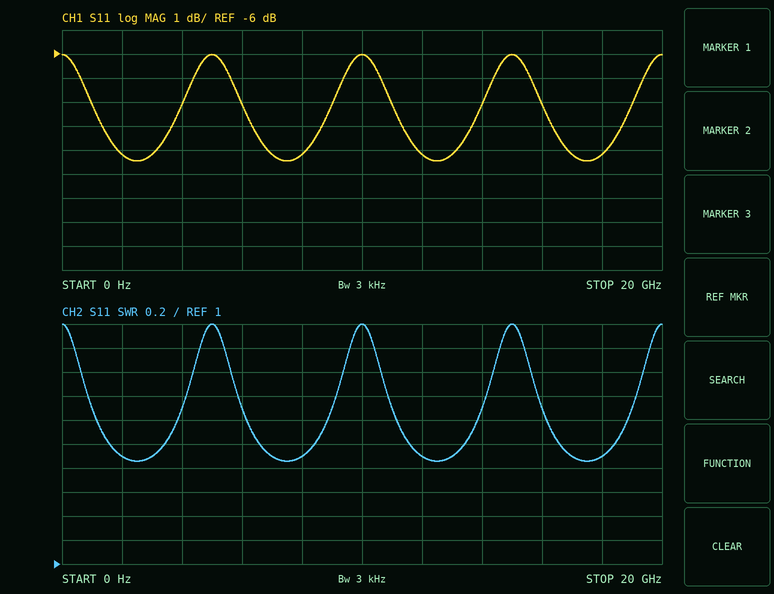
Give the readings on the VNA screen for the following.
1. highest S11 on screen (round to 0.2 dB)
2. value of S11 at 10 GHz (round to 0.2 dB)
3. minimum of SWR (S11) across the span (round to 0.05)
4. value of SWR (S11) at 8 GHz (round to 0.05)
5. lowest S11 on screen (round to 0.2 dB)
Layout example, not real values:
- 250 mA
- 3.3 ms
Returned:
- -6.0 dB
- -6.0 dB
- 1.85
- 1.90
- -10.4 dB
